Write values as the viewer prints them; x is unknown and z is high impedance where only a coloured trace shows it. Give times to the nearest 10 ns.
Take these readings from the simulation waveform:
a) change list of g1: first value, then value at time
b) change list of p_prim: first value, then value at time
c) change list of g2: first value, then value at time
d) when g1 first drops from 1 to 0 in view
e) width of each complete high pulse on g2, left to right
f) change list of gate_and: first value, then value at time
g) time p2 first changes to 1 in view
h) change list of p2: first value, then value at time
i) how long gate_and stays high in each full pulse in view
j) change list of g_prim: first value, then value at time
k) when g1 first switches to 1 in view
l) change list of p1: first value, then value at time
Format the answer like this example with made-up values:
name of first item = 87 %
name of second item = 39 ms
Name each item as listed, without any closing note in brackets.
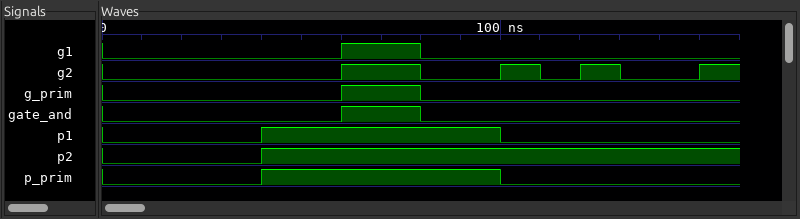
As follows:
change list of g1: first value, then value at time = 0, 1 at 60 ns, 0 at 80 ns
change list of p_prim: first value, then value at time = 0, 1 at 40 ns, 0 at 100 ns
change list of g2: first value, then value at time = 0, 1 at 60 ns, 0 at 80 ns, 1 at 100 ns, 0 at 110 ns, 1 at 120 ns, 0 at 130 ns, 1 at 150 ns
when g1 first drops from 1 to 0 in view = 80 ns
width of each complete high pulse on g2, left to right = 20 ns, 10 ns, 10 ns
change list of gate_and: first value, then value at time = 0, 1 at 60 ns, 0 at 80 ns
time p2 first changes to 1 in view = 40 ns
change list of p2: first value, then value at time = 0, 1 at 40 ns
how long gate_and stays high in each full pulse in view = 20 ns
change list of g_prim: first value, then value at time = 0, 1 at 60 ns, 0 at 80 ns
when g1 first switches to 1 in view = 60 ns
change list of p1: first value, then value at time = 0, 1 at 40 ns, 0 at 100 ns
